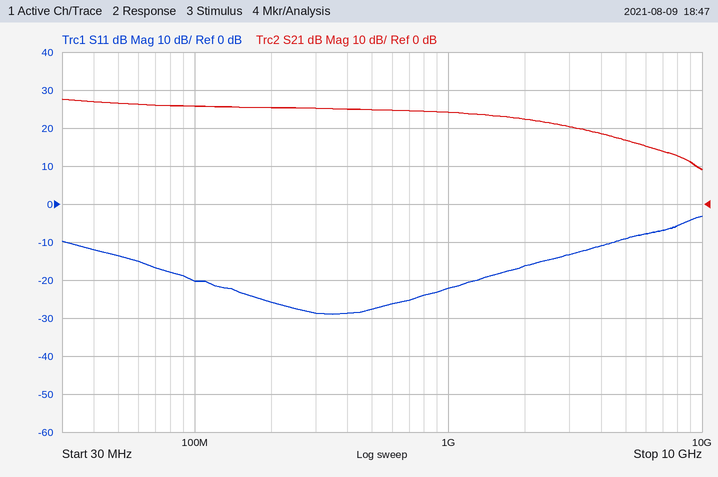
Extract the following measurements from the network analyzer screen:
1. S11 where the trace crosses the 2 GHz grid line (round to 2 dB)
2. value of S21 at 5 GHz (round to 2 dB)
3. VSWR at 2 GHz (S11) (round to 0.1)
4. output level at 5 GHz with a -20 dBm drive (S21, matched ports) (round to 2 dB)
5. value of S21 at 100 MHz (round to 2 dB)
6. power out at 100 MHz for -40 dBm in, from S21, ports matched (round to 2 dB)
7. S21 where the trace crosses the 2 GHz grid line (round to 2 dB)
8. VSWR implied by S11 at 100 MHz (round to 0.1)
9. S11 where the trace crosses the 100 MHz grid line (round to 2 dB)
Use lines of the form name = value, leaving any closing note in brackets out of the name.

S11 where the trace crosses the 2 GHz grid line = -16 dB
value of S21 at 5 GHz = 16 dB
VSWR at 2 GHz (S11) = 1.4
output level at 5 GHz with a -20 dBm drive (S21, matched ports) = -4 dBm
value of S21 at 100 MHz = 26 dB
power out at 100 MHz for -40 dBm in, from S21, ports matched = -14 dBm
S21 where the trace crosses the 2 GHz grid line = 22 dB
VSWR implied by S11 at 100 MHz = 1.2
S11 where the trace crosses the 100 MHz grid line = -20 dB
